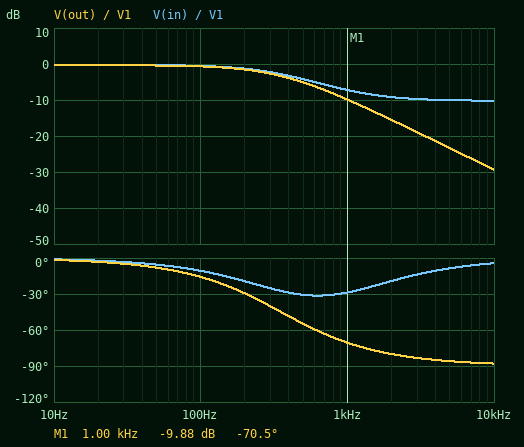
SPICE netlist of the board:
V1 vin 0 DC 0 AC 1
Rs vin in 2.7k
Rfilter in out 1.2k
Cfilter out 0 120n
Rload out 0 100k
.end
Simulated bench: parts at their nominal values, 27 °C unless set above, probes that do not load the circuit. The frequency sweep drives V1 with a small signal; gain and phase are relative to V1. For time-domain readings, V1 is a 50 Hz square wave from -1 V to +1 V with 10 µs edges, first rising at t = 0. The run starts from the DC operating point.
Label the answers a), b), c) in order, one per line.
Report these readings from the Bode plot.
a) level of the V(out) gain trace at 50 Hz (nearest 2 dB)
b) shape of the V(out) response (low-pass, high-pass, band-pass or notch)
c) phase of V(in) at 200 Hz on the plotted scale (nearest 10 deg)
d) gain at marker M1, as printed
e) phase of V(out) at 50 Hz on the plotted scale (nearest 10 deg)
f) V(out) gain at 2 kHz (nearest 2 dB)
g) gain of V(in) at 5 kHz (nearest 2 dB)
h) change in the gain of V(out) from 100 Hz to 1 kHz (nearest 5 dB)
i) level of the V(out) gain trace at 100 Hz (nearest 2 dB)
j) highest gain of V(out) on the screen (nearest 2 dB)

a) 0 dB
b) low-pass
c) -20 deg
d) -9.88 dB
e) -10 deg
f) -16 dB
g) -10 dB
h) -10 dB
i) 0 dB
j) 0 dB
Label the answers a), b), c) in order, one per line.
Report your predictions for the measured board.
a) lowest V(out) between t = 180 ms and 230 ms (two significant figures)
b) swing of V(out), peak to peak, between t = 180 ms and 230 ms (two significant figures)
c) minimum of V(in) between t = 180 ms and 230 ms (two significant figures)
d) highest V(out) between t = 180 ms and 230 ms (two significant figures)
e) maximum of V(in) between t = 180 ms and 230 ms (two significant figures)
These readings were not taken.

a) -960 mV
b) 1.9 V
c) -970 mV
d) 960 mV
e) 970 mV
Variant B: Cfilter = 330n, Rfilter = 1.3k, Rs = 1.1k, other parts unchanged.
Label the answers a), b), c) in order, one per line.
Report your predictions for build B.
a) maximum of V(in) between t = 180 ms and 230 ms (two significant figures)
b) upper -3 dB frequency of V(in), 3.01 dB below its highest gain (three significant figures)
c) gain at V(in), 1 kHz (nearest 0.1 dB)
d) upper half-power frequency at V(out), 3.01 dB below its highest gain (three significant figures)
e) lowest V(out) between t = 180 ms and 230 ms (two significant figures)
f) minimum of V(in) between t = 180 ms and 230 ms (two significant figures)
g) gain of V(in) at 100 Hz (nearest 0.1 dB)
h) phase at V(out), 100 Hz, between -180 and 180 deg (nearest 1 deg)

a) 990 mV
b) 325 Hz
c) -4.9 dB
d) 206 Hz
e) -980 mV
f) -990 mV
g) -0.7 dB
h) -26 deg
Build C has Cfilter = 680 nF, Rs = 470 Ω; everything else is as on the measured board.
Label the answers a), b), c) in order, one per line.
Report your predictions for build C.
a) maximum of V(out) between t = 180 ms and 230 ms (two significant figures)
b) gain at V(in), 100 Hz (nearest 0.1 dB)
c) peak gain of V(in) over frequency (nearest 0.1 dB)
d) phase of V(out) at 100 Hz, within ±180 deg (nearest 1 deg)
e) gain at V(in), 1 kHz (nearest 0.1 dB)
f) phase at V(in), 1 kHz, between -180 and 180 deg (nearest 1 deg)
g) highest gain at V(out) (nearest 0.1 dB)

a) 980 mV
b) -0.8 dB
c) 0 dB
d) -35 deg
e) -2.8 dB
f) -3 deg
g) -0.1 dB
